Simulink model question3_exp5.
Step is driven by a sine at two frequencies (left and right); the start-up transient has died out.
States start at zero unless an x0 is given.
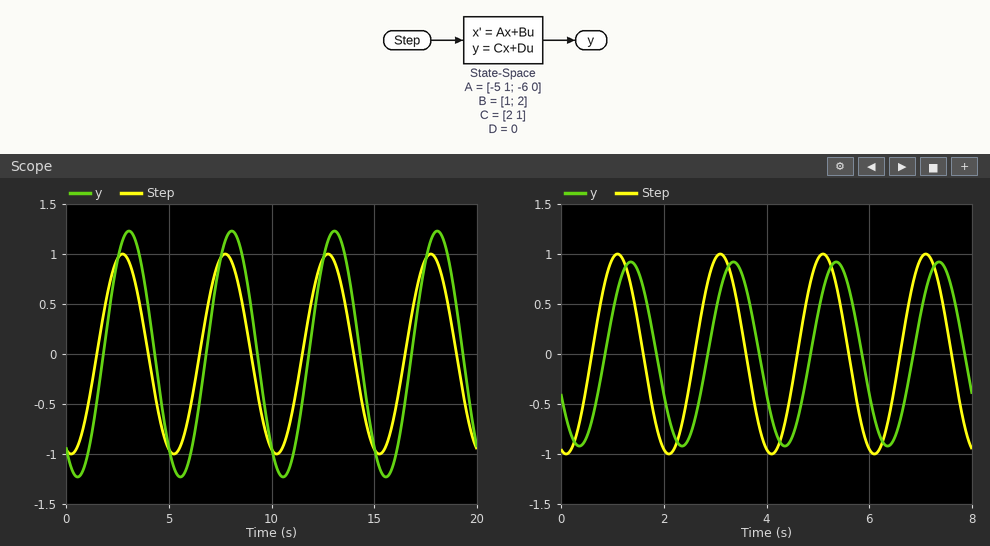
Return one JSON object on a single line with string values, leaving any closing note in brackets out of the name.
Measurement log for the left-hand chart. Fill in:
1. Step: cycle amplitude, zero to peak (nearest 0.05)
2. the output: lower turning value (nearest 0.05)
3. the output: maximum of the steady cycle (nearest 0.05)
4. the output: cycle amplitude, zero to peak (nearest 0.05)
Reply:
{"Step: cycle amplitude, zero to peak": "1.00", "the output: lower turning value": "-1.25", "the output: maximum of the steady cycle": "1.25", "the output: cycle amplitude, zero to peak": "1.25"}
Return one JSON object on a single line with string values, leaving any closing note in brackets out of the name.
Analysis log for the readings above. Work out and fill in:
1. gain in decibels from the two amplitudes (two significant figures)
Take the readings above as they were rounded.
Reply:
{"gain in decibels from the two amplitudes": "1.9 dB"}
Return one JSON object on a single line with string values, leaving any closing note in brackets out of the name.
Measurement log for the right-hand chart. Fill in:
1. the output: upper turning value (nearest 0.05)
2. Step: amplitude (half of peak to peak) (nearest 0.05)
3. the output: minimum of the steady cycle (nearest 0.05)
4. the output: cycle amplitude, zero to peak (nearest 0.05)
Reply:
{"the output: upper turning value": "0.90", "Step: amplitude (half of peak to peak)": "1.00", "the output: minimum of the steady cycle": "-0.90", "the output: cycle amplitude, zero to peak": "0.90"}
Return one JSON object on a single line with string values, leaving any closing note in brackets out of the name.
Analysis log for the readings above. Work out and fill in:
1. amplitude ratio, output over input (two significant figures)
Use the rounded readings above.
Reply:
{"amplitude ratio, output over input": "0.90"}
